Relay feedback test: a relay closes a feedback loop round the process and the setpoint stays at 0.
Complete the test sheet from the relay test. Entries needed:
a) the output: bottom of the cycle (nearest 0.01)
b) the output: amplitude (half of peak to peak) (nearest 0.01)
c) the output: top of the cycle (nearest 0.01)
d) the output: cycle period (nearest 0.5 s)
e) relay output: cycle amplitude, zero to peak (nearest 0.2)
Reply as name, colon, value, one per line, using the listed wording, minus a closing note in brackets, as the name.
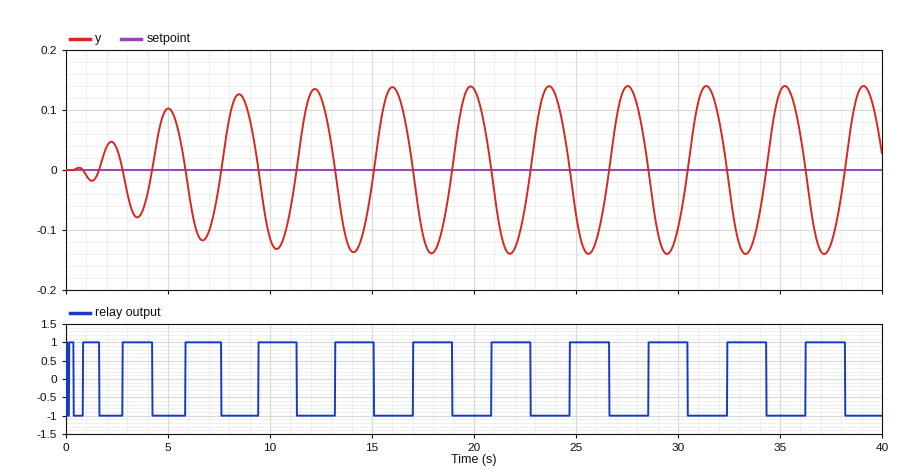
the output: bottom of the cycle: -0.14
the output: amplitude (half of peak to peak): 0.14
the output: top of the cycle: 0.14
the output: cycle period: 4.0 s
relay output: cycle amplitude, zero to peak: 1.0
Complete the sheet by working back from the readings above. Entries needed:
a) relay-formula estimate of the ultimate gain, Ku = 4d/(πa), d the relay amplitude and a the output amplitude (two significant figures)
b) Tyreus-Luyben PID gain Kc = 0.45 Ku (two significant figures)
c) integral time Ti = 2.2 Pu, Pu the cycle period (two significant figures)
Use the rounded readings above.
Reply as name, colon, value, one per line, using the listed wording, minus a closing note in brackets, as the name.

relay-formula estimate of the ultimate gain, Ku = 4d/(πa), d the relay amplitude and a the output amplitude: 9.1
Tyreus-Luyben PID gain Kc = 0.45 Ku: 4.1
integral time Ti = 2.2 Pu, Pu the cycle period: 8.8 s
